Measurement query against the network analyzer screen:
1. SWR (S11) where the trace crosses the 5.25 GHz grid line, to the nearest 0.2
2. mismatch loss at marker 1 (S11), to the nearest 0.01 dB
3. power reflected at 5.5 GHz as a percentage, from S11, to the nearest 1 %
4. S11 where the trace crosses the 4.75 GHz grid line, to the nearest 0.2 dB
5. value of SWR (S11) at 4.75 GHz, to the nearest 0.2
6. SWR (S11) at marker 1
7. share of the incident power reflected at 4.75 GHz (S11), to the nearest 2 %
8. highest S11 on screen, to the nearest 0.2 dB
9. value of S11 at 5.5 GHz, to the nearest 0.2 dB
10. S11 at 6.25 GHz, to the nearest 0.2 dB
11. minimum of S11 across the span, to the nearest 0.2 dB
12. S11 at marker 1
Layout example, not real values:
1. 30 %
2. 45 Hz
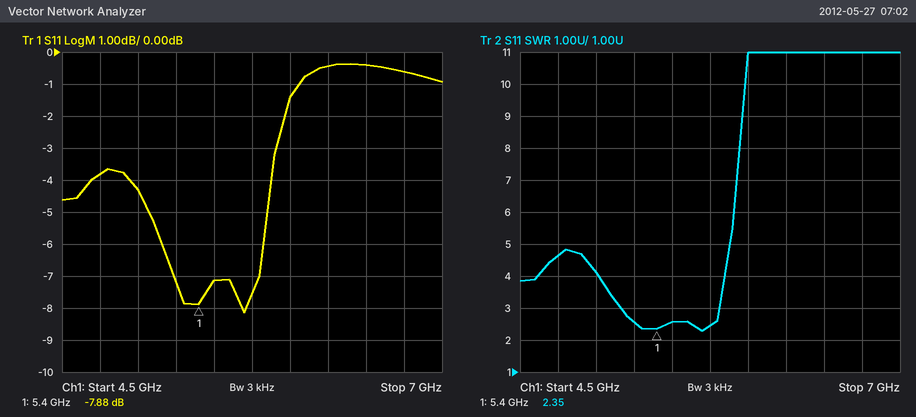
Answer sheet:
1. 2.6
2. 0.77 dB
3. 19 %
4. -3.8 dB
5. 4.6
6. 2.35
7. 42 %
8. -0.4 dB
9. -7.2 dB
10. -0.4 dB
11. -8.2 dB
12. -7.88 dB
